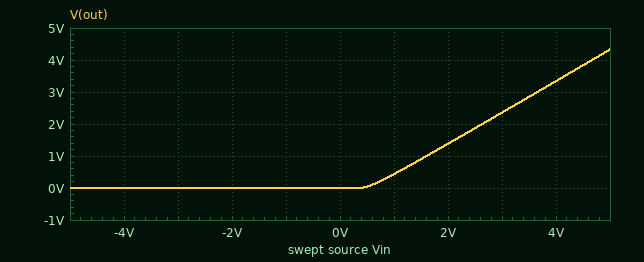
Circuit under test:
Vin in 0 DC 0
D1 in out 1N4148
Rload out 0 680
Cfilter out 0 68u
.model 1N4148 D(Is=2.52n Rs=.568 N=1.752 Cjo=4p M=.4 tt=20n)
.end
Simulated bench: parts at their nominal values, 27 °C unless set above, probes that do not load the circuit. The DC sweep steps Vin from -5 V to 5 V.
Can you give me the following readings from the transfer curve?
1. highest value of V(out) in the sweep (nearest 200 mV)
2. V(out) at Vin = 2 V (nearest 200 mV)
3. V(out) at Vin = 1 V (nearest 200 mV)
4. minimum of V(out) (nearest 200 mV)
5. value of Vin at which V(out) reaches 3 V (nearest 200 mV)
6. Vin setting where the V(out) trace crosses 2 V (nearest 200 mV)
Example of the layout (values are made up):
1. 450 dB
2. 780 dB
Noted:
1. 4.4 V
2. 1.4 V
3. 400 mV
4. 0 V
5. 3.6 V
6. 2.6 V
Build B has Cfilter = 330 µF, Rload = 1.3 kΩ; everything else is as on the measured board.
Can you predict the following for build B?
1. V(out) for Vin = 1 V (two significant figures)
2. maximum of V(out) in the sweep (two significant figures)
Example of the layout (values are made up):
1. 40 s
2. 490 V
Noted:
1. 460 mV
2. 4.4 V
